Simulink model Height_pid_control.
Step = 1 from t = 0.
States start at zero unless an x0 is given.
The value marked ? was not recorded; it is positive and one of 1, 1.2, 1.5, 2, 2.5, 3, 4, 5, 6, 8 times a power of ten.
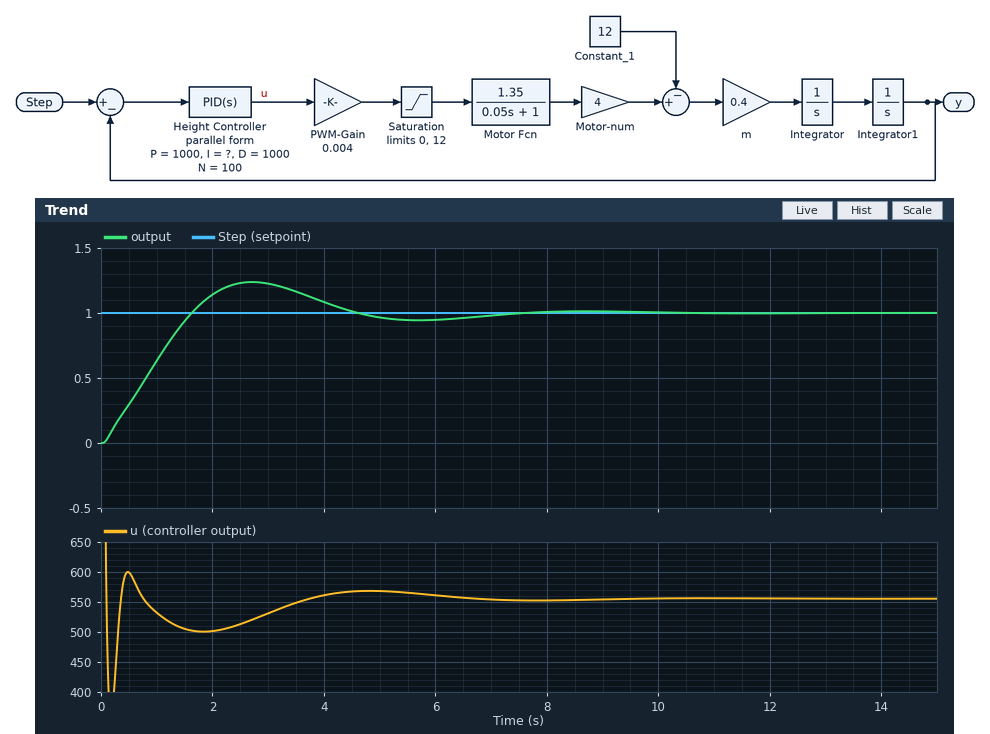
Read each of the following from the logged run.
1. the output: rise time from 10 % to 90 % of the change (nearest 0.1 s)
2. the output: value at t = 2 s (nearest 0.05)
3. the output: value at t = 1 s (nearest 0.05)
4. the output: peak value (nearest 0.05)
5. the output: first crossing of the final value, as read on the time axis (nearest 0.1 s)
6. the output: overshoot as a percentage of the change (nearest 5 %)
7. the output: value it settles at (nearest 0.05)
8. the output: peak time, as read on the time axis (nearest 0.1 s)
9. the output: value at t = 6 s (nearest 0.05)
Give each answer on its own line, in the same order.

1.2 s
1.15
0.65
1.25
1.6 s
25 %
1.00
2.7 s
0.95
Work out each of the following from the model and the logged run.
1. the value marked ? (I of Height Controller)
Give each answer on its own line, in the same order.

1200
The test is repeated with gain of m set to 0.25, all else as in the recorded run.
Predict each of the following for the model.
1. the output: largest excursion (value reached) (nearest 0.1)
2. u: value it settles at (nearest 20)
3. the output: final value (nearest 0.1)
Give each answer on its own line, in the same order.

1.3
560
1.0
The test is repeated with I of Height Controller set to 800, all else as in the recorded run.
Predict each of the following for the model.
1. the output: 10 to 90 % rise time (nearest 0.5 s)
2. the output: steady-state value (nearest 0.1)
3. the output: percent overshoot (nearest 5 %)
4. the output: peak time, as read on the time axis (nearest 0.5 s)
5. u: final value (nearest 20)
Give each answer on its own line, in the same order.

1.5 s
1.0
15 %
3.5 s
560
